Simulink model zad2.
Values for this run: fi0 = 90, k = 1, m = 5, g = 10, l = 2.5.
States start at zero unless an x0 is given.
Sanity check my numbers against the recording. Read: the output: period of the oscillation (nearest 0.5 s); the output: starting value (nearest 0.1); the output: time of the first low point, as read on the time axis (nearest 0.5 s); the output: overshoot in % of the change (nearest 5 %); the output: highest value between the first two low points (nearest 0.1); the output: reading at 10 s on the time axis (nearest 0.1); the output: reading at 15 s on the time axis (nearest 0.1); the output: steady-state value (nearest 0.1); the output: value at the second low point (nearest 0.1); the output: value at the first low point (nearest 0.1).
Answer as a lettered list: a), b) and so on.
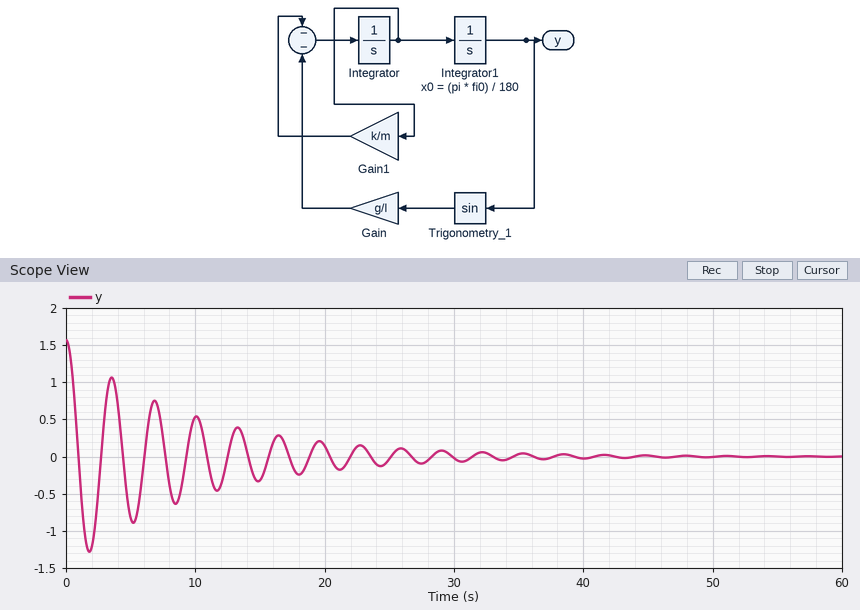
a) 3.5 s
b) 1.6
c) 2.0 s
d) 80 %
e) 1.1
f) 0.5
g) -0.3
h) 0.0
i) -0.9
j) -1.3
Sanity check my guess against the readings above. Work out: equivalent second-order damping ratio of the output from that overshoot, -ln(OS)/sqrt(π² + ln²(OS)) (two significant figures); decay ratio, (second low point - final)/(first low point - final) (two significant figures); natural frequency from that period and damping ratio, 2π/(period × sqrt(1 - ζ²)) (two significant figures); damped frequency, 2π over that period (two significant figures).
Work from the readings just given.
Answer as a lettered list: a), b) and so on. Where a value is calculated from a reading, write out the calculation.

a) ln(0.8) = -0.223; 0.223 / sqrt(9.870 + 0.050) = 0.071
b) (-0.9 - 0) / (-1.3 - 0) = 0.69
c) 2π / (3.5 × sqrt(1 - 0.071²)) = 1.8 rad/s
d) 2π / 3.5 = 1.8 rad/s
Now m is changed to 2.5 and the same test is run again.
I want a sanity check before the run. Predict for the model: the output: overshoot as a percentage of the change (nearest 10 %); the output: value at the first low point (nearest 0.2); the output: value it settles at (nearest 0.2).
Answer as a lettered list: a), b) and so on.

a) 70 %
b) -1.0
c) 0.0
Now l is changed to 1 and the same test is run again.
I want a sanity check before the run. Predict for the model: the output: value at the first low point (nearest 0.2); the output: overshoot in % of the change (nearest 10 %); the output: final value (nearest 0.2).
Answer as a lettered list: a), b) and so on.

a) -1.4
b) 90 %
c) 0.0
